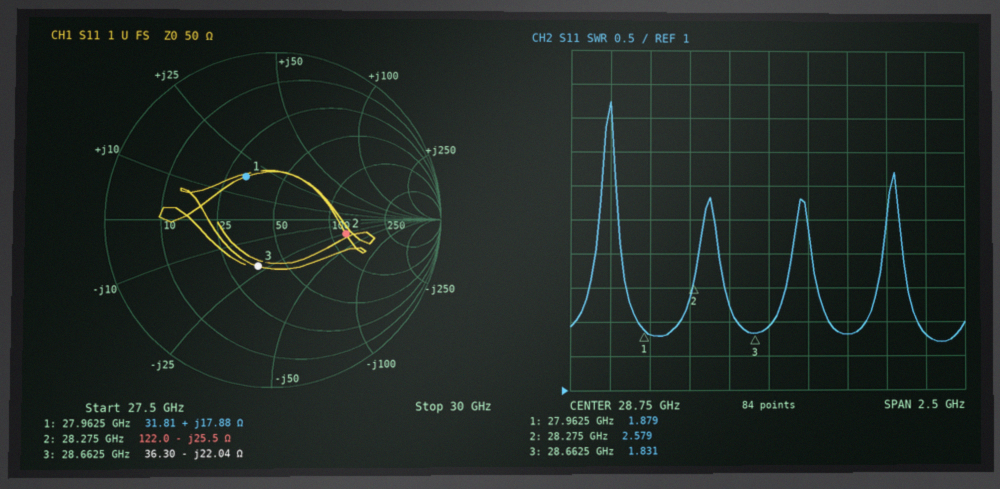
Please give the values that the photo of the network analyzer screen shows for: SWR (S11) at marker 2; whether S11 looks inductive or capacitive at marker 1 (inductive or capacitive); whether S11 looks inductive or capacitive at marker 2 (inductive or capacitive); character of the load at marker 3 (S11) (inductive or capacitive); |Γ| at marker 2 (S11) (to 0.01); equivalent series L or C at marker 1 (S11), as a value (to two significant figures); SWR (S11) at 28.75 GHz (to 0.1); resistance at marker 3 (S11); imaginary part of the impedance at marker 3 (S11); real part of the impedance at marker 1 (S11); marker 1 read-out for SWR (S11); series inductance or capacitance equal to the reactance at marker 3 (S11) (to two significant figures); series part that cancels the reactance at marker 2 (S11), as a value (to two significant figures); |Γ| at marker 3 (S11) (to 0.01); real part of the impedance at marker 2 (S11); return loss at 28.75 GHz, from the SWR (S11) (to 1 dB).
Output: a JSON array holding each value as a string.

["2.579", "inductive", "capacitive", "capacitive", "0.44", "100 pH", "1.9", "36.30 Ω", "-22.04 Ω", "31.81 Ω", "1.879", "250 fF", "140 pH", "0.29", "122.0 Ω", "10 dB"]
